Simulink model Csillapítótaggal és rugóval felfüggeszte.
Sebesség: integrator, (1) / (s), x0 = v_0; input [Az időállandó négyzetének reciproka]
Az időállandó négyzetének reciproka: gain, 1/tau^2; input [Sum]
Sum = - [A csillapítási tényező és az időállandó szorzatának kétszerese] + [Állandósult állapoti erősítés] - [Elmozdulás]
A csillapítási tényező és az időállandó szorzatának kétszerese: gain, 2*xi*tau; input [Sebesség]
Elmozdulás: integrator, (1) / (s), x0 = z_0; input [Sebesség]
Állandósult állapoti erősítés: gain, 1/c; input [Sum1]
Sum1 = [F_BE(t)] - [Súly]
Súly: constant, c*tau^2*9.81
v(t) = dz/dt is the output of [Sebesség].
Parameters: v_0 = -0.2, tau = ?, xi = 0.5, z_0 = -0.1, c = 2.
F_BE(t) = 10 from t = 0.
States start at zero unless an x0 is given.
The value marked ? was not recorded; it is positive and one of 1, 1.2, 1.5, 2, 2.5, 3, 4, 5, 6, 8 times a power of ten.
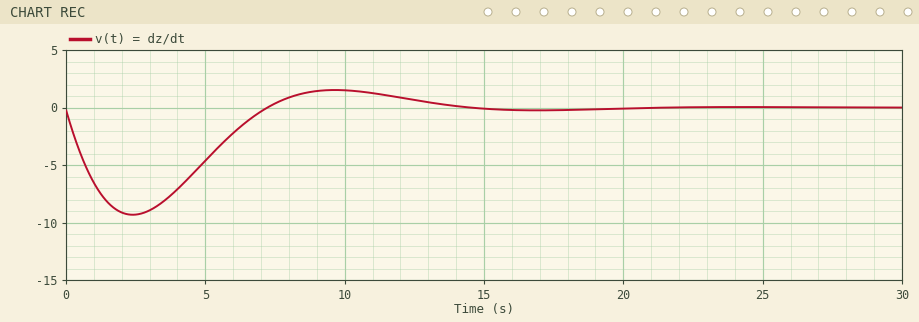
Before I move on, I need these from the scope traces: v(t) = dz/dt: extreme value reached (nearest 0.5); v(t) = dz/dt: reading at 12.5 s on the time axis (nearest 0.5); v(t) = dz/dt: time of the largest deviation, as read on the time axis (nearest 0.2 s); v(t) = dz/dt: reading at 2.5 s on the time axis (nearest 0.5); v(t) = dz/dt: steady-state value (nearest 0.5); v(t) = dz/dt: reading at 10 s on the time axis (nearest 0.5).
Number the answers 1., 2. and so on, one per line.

1. -9.5
2. 0.5
3. 2.4 s
4. -9.5
5. 0.0
6. 1.5
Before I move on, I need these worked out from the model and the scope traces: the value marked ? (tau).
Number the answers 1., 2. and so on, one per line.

1. 2
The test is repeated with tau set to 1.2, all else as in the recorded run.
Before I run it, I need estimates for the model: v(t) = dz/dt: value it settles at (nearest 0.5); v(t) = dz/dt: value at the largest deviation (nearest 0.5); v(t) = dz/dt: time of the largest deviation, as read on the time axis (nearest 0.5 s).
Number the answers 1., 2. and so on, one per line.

1. 0.0
2. -4.0
3. 1.5 s
